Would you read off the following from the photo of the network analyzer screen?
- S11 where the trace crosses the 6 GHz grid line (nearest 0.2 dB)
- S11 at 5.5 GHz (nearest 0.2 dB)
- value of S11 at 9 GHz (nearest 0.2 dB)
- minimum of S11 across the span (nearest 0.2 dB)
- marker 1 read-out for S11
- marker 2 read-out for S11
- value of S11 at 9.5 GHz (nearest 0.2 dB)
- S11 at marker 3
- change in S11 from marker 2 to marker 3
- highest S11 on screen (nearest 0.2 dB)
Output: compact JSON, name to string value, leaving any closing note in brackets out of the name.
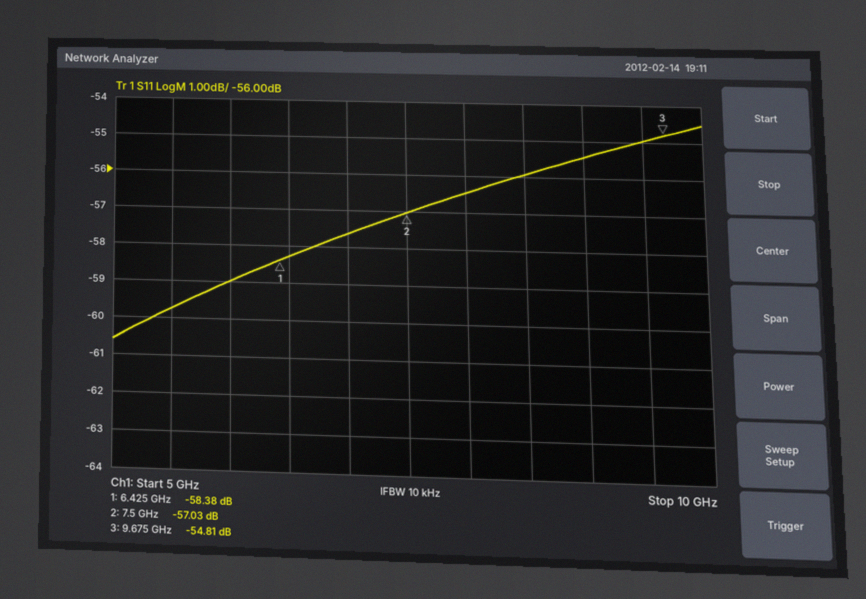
{"S11 where the trace crosses the 6 GHz grid line": "-59.0 dB", "S11 at 5.5 GHz": "-59.8 dB", "value of S11 at 9 GHz": "-55.4 dB", "minimum of S11 across the span": "-60.6 dB", "marker 1 read-out for S11": "-58.38 dB", "marker 2 read-out for S11": "-57.03 dB", "value of S11 at 9.5 GHz": "-55.0 dB", "S11 at marker 3": "-54.81 dB", "change in S11 from marker 2 to marker 3": "2.22 dB", "highest S11 on screen": "-54.6 dB"}
